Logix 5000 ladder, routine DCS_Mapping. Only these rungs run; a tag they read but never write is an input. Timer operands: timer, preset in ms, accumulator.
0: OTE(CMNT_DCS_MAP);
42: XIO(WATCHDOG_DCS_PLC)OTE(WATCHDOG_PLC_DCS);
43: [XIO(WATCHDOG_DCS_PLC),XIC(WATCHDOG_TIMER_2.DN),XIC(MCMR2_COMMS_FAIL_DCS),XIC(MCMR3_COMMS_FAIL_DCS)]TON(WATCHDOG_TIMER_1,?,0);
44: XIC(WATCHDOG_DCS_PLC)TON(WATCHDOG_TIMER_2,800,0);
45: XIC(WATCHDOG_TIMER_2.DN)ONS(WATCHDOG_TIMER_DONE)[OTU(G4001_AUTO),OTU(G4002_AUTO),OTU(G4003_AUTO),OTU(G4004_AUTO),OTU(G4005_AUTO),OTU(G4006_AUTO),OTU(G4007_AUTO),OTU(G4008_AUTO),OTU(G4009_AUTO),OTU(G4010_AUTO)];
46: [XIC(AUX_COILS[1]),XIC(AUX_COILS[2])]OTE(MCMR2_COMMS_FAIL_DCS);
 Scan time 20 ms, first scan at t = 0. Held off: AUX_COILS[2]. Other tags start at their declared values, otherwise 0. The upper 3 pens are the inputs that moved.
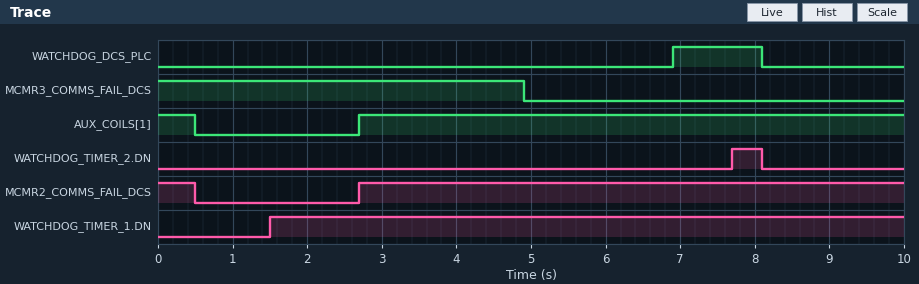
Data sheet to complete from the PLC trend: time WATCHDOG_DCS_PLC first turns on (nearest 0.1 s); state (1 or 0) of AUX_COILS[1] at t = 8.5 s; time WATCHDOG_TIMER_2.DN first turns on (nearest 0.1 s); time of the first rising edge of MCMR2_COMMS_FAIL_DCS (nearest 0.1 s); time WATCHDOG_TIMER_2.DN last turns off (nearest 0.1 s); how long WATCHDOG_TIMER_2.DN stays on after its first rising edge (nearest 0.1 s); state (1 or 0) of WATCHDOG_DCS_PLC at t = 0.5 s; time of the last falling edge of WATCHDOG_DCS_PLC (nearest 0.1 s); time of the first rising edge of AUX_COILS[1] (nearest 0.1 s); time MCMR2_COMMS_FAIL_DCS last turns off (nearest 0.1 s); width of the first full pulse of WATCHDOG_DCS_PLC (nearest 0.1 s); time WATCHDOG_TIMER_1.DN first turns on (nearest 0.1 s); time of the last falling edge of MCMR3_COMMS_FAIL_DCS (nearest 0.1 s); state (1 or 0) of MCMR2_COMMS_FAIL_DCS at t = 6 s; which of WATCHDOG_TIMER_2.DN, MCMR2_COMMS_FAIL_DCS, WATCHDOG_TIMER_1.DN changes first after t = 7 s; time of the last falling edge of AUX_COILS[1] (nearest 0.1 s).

6.9 s
1
7.7 s
2.7 s
8.1 s
0.4 s
0
8.1 s
2.7 s
0.5 s
1.2 s
1.5 s
4.9 s
1
WATCHDOG_TIMER_2.DN
0.5 s
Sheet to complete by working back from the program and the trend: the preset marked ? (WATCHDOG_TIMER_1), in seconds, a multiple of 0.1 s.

1.5 s
